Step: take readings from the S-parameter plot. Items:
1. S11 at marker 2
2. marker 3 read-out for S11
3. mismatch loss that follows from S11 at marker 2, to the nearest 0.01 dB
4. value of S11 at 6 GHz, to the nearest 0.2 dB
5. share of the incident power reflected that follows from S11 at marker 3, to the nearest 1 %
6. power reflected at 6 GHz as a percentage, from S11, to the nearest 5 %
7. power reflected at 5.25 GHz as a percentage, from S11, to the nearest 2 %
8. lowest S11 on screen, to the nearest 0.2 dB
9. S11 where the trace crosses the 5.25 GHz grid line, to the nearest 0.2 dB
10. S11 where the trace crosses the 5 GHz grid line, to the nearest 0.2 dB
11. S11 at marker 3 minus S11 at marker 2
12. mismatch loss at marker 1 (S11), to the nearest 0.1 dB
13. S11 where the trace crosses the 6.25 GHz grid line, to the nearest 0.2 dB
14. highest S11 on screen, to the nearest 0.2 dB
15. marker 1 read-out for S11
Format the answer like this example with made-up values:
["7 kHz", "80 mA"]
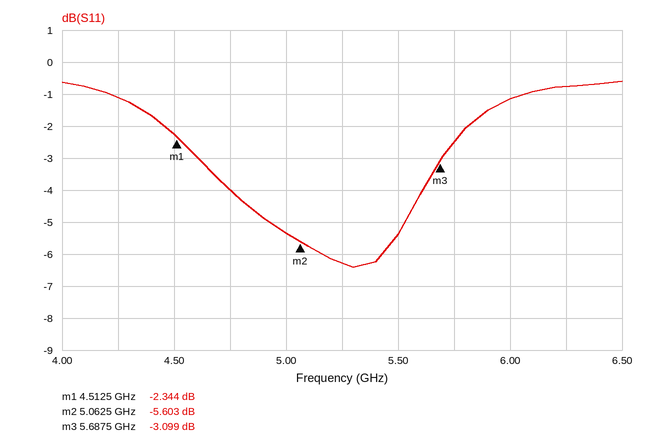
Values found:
["-5.603 dB", "-3.099 dB", "1.40 dB", "-1.2 dB", "49 %", "75 %", "24 %", "-6.4 dB", "-6.2 dB", "-5.4 dB", "2.504 dB", "3.8 dB", "-0.8 dB", "-0.6 dB", "-2.344 dB"]
